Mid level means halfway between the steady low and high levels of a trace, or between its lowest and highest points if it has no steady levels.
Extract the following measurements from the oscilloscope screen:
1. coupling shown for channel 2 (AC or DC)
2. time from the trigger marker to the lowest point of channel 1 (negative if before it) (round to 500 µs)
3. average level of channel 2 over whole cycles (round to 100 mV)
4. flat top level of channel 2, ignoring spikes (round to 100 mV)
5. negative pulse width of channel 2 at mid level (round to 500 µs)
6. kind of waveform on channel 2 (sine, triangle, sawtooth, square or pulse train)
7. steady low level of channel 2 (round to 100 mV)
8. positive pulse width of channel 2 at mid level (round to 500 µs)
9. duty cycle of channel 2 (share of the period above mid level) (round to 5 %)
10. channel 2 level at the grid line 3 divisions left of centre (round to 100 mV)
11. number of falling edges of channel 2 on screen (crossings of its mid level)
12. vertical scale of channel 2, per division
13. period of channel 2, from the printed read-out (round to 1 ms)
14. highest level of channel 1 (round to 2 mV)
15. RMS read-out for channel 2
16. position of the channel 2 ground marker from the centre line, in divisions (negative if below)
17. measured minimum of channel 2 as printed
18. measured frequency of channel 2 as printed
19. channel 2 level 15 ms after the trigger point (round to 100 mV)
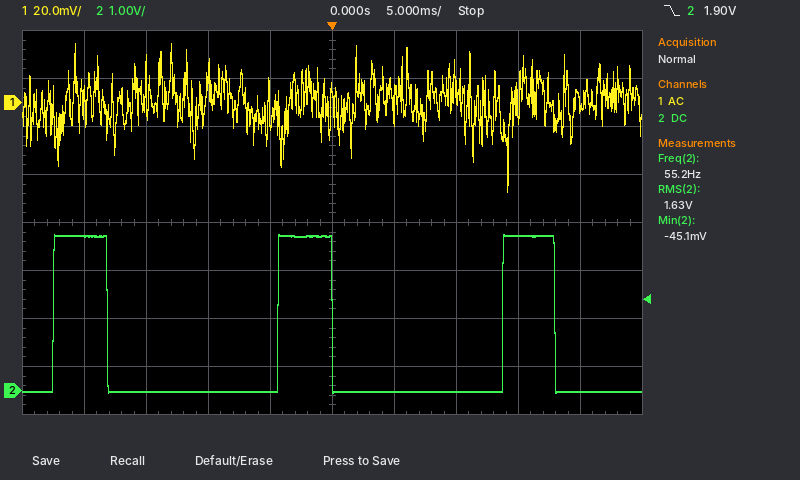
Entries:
DC
+14.0 ms
800 mV
3.2 V
14.0 ms
pulse train
0.0 V
4.5 ms
25 %
0.0 V
3
1 V
18 ms
24 mV
1.63 V
-3.5 div
-45.1 mV
55.2 Hz
3.2 V
